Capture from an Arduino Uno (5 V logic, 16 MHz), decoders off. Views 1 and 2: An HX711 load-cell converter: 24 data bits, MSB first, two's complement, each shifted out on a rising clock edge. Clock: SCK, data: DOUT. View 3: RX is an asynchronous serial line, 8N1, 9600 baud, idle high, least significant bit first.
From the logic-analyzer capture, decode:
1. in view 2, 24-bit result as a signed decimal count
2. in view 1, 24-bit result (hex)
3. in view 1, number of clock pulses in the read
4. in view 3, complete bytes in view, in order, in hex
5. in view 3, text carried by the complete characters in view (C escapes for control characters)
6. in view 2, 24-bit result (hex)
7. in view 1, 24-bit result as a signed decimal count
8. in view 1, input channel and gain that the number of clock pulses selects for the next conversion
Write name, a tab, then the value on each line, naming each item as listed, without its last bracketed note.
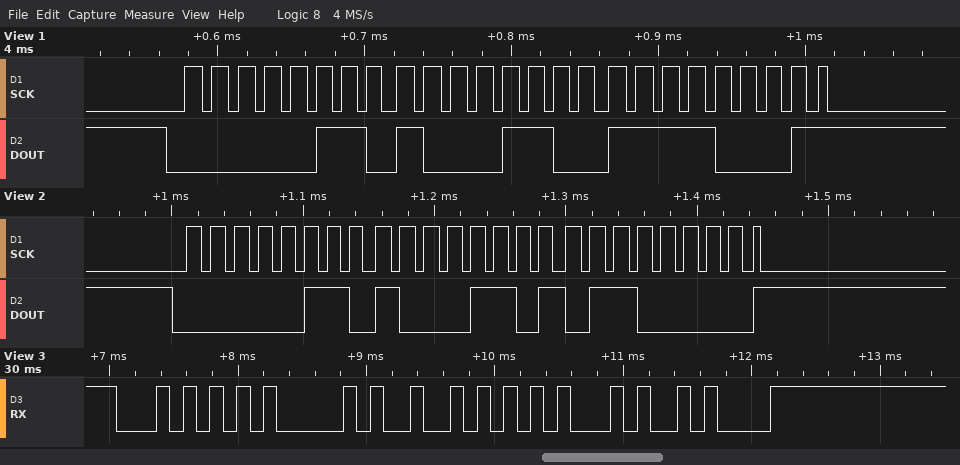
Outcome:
in view 2, 24-bit result as a signed decimal count	429408
in view 1, 24-bit result	0x068CF1
in view 1, number of clock pulses in the read	25
in view 3, complete bytes in view, in order, in hex	0x54 0x41 0x52 0x45 0x0A
in view 3, text carried by the complete characters in view	"TARE\n"
in view 2, 24-bit result	0x068D60
in view 1, 24-bit result as a signed decimal count	429297
in view 1, input channel and gain that the number of clock pulses selects for the next conversion	channel A, gain 128
